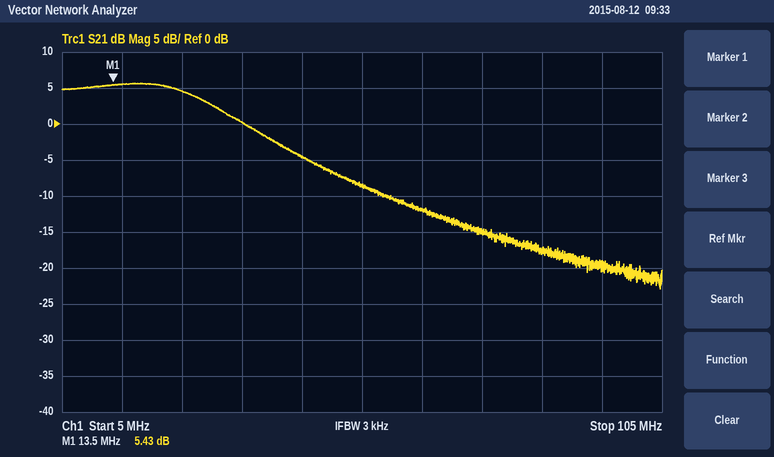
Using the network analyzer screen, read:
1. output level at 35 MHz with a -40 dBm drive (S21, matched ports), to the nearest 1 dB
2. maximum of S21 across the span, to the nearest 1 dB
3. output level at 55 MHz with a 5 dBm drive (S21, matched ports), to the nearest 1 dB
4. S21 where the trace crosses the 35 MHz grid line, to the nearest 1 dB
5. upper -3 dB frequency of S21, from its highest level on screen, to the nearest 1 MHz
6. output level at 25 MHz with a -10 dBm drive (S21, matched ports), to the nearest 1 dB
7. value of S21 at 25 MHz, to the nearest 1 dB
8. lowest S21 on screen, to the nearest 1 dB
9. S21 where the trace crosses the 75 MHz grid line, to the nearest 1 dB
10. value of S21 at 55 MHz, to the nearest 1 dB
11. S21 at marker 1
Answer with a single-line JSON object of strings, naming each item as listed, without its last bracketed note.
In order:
{"output level at 35 MHz with a -40 dBm drive (S21, matched ports), to the nearest 1 dB": "-40 dBm", "maximum of S21 across the span, to the nearest 1 dB": "6 dB", "output level at 55 MHz with a 5 dBm drive (S21, matched ports), to the nearest 1 dB": "-4 dBm", "S21 where the trace crosses the 35 MHz grid line, to the nearest 1 dB": "0 dB", "upper -3 dB frequency of S21, from its highest level on screen, to the nearest 1 MHz": "30 MHz", "output level at 25 MHz with a -10 dBm drive (S21, matched ports), to the nearest 1 dB": "-5 dBm", "value of S21 at 25 MHz, to the nearest 1 dB": "5 dB", "lowest S21 on screen, to the nearest 1 dB": "-23 dB", "S21 where the trace crosses the 75 MHz grid line, to the nearest 1 dB": "-15 dB", "value of S21 at 55 MHz, to the nearest 1 dB": "-9 dB", "S21 at marker 1": "5.43 dB"}
